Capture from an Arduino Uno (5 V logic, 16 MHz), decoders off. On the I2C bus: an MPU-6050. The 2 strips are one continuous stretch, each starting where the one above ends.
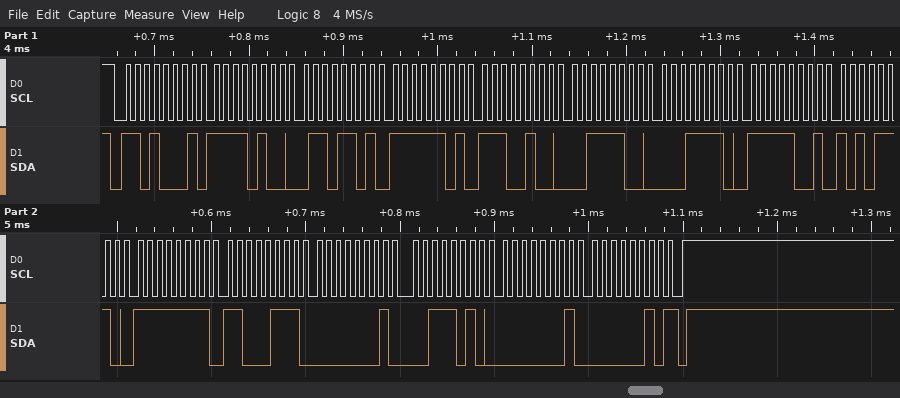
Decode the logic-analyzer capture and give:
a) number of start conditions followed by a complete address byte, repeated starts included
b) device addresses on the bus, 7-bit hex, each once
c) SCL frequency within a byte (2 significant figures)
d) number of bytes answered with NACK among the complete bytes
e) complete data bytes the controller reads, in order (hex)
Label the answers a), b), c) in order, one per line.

a) 1
b) 0x68
c) 100 kHz
d) 1
e) F4 6D FD E4 3C 1E F9 AE FF C7 01 3A 01 02
